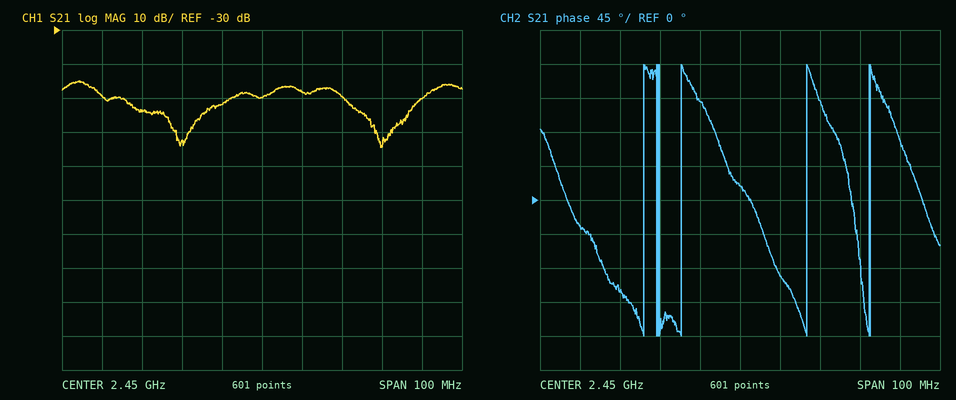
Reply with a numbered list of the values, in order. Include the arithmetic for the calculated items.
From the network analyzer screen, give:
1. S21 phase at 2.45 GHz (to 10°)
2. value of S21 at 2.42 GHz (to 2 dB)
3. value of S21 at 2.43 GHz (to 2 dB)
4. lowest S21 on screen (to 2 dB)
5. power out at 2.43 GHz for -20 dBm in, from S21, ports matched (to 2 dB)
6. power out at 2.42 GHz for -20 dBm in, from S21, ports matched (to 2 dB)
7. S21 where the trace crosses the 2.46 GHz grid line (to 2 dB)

1. 20°
2. -54 dB
3. -62 dB
4. -64 dB
5. -20 dBm + (-62 dB) = -82 dBm
6. -20 dBm + (-54 dB) = -74 dBm
7. -48 dB
